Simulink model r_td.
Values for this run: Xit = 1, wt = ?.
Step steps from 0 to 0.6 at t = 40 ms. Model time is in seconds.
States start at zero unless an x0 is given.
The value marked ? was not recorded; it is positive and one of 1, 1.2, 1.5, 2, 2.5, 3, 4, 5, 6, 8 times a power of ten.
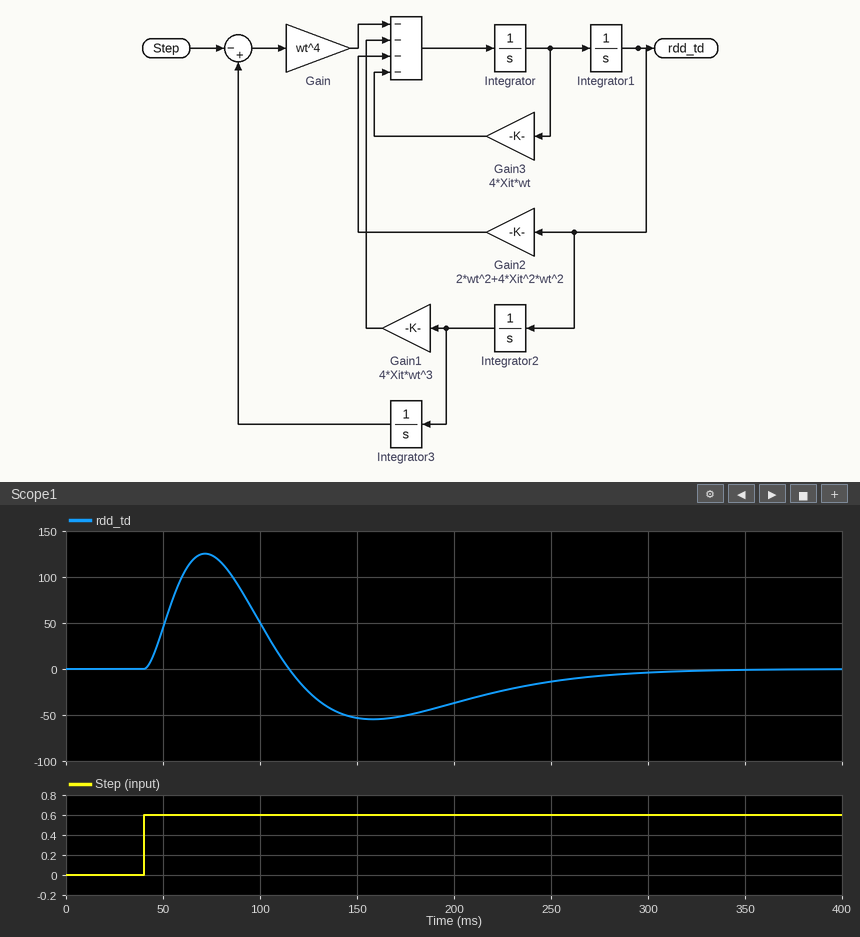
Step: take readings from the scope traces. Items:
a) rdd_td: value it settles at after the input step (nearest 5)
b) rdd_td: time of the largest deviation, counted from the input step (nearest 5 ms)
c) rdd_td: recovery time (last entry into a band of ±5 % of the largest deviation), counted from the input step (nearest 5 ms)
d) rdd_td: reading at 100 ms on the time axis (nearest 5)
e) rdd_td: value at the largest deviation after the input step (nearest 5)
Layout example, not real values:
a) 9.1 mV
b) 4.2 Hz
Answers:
a) 0
b) 30 ms
c) 240 ms
d) 50
e) 125
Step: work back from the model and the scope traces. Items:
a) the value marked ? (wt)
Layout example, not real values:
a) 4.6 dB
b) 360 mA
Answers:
a) 40
